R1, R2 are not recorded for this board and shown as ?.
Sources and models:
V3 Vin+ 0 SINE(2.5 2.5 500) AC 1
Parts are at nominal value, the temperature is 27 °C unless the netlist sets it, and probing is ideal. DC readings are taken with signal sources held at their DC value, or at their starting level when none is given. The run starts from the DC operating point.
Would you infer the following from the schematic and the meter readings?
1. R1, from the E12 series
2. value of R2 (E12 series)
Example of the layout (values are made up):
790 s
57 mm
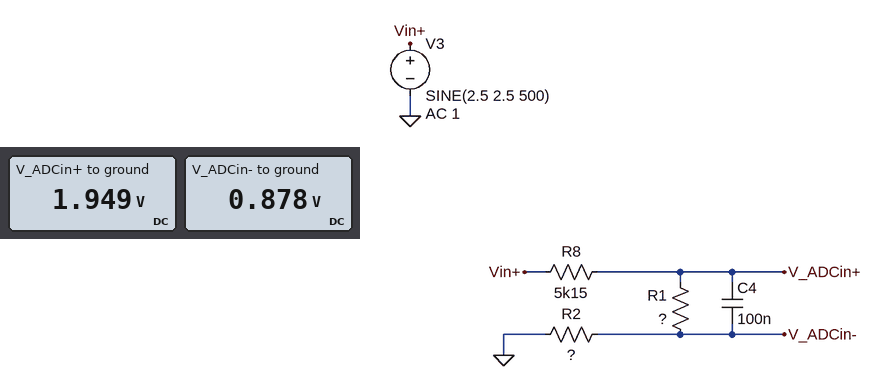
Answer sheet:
10 kΩ
8.2 kΩ
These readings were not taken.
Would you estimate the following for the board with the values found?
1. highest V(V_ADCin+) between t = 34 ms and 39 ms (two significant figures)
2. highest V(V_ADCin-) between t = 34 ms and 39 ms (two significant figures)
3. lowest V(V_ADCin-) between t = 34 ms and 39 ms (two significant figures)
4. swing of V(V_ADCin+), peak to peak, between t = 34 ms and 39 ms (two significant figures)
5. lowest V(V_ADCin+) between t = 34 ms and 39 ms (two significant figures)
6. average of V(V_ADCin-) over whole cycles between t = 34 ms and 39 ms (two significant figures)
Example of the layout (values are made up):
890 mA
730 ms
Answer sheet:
3.6 V
2.3 V
-530 mV
3.3 V
310 mV
880 mV
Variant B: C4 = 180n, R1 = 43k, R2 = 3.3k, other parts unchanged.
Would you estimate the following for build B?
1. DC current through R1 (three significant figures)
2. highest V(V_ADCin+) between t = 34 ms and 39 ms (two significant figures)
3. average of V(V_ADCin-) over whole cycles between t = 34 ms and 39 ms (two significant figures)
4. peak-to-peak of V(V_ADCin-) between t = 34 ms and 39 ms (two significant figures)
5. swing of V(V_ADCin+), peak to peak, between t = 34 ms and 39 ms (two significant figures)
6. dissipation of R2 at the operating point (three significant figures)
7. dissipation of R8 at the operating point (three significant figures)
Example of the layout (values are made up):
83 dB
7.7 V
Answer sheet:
48.6 µA
3.3 V
160 mV
1.9 V
2.2 V
7.79 µW
12.2 µW
